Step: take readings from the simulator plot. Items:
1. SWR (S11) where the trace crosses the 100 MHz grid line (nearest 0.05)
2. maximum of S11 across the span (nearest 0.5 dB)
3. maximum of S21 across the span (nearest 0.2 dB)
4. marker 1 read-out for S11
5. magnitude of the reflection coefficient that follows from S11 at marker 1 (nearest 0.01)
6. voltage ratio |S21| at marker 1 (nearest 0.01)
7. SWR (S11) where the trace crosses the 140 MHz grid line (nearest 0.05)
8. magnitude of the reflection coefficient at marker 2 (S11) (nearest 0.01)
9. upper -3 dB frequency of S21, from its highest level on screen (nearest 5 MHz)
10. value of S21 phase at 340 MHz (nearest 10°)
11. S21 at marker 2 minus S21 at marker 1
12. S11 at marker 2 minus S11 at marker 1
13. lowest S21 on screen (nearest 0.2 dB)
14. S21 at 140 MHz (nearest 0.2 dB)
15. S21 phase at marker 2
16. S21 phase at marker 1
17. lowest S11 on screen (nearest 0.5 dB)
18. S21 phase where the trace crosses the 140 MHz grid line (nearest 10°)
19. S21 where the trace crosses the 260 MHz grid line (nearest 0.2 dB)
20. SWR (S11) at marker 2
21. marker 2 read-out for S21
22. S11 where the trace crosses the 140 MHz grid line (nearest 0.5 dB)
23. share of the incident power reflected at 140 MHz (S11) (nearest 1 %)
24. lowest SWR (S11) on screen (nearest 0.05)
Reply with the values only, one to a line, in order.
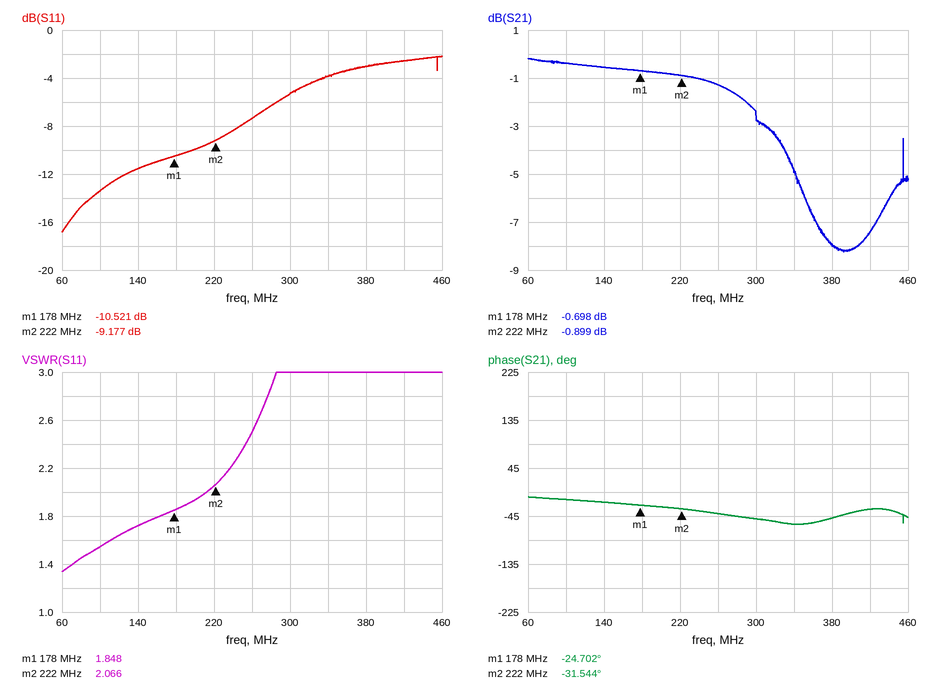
1.55
-2.0 dB
-0.2 dB
-10.521 dB
0.30
0.92
1.70
0.35
315 MHz
-60°
-0.201 dB
1.344 dB
-8.2 dB
-0.6 dB
-31.544°
-24.702°
-17.0 dB
-20°
-1.2 dB
2.066
-0.899 dB
-11.5 dB
7 %
1.35
